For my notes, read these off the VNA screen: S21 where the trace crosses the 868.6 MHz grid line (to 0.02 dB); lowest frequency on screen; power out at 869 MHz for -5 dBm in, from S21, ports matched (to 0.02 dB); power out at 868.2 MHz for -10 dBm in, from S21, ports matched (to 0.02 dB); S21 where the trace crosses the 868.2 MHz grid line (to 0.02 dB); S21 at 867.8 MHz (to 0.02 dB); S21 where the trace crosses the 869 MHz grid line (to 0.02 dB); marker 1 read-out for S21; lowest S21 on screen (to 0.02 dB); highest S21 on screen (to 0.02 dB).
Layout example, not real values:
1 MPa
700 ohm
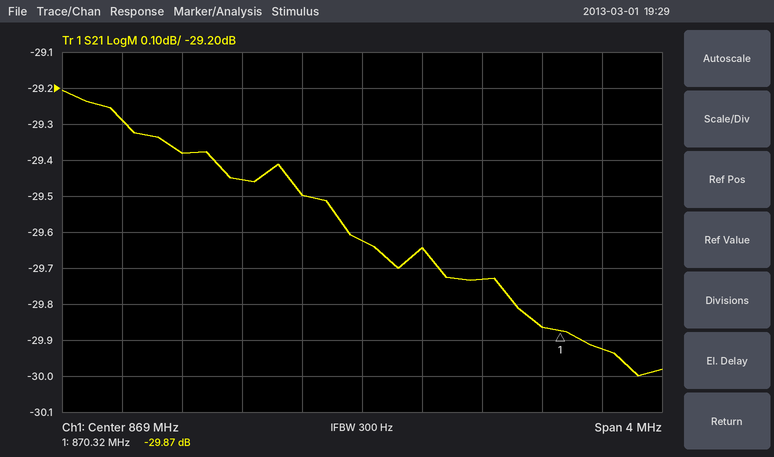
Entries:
-29.50 dB
867 MHz
-34.62 dBm
-39.46 dBm
-29.46 dB
-29.38 dB
-29.62 dB
-29.87 dB
-30.00 dB
-29.20 dB
